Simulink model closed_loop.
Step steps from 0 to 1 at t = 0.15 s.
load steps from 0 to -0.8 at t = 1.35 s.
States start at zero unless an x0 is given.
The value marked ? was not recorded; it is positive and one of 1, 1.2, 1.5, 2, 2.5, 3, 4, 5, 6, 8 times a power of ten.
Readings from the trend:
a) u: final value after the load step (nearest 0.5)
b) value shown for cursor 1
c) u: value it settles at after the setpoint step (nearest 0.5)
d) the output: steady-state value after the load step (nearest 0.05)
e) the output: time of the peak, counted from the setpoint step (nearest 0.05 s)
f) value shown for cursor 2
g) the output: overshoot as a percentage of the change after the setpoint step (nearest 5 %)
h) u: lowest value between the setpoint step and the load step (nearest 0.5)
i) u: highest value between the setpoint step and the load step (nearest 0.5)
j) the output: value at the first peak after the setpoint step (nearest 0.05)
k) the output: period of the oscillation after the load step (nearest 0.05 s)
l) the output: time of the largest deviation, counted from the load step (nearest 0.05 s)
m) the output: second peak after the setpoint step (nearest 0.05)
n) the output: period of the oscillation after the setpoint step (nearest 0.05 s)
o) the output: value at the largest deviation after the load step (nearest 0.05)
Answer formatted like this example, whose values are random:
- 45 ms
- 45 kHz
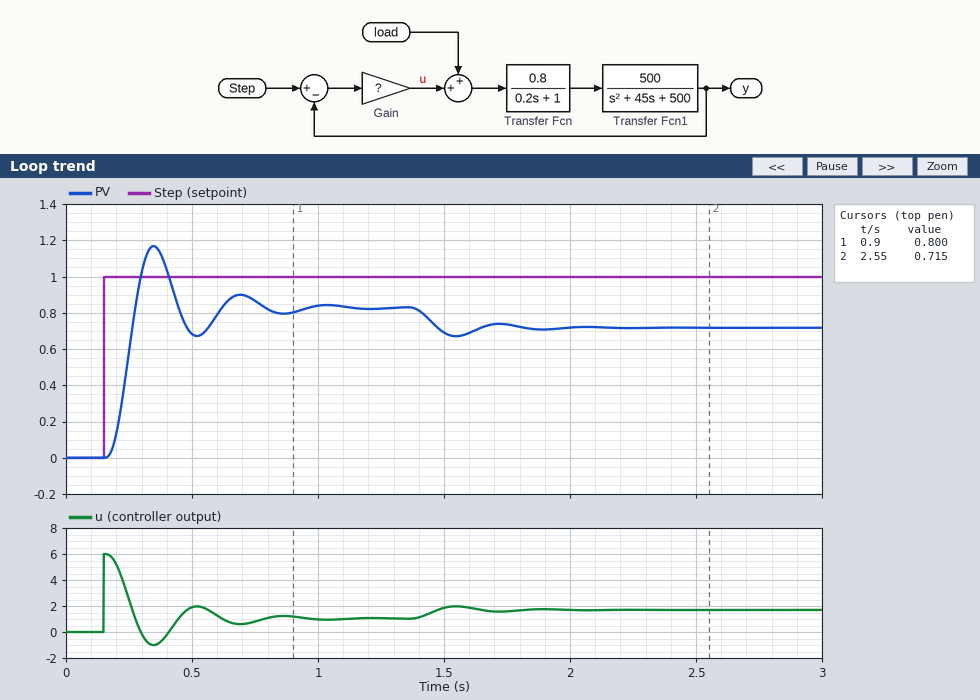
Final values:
- 1.5
- 0.800
- 1.0
- 0.70
- 0.20 s
- 0.715
- 40 %
- -1.0
- 6.0
- 1.15
- 0.35 s
- 0.20 s
- 0.90
- 0.35 s
- 0.65
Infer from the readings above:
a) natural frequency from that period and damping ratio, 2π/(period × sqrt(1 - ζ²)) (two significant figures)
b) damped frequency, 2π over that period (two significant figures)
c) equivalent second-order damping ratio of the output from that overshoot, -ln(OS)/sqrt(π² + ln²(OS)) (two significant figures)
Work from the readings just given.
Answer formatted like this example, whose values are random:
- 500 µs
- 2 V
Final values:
- 19 rad/s
- 18 rad/s
- 0.28
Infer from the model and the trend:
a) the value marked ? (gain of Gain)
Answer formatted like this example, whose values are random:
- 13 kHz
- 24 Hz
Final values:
- 6
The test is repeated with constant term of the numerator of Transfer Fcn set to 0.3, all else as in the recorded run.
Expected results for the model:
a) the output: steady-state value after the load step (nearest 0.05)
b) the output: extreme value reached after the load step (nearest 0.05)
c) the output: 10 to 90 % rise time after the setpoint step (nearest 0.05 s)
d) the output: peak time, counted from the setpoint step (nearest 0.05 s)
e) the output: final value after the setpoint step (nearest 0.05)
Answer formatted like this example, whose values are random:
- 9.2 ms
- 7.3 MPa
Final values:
- 0.55
- 0.55
- 0.15 s
- 0.30 s
- 0.65
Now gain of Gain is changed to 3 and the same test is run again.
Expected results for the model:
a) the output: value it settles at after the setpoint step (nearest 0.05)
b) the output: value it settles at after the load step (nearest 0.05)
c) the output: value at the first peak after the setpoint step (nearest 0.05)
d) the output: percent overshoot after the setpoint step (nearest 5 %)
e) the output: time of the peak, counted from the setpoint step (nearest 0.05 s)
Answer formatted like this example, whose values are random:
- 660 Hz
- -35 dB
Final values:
- 0.70
- 0.50
- 0.85
- 20 %
- 0.25 s
